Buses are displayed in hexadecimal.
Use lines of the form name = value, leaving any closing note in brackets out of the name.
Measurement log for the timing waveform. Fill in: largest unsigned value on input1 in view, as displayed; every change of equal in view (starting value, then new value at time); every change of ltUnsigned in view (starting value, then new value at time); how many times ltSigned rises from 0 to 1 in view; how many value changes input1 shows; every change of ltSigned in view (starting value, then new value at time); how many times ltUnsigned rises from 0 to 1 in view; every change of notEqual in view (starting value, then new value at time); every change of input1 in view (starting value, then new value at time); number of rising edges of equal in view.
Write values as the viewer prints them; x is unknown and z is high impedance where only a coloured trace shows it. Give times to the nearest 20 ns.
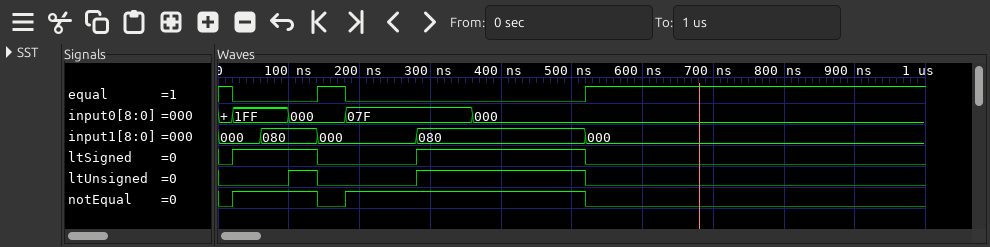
largest unsigned value on input1 in view, as displayed = 080
every change of equal in view = 1, 0 at 20 ns, 1 at 140 ns, 0 at 180 ns, 1 at 520 ns
every change of ltUnsigned in view = 0, 1 at 100 ns, 0 at 140 ns, 1 at 280 ns, 0 at 520 ns
how many times ltSigned rises from 0 to 1 in view = 2
how many value changes input1 shows = 4
every change of ltSigned in view = 0, 1 at 20 ns, 0 at 140 ns, 1 at 280 ns, 0 at 520 ns
how many times ltUnsigned rises from 0 to 1 in view = 2
every change of notEqual in view = 0, 1 at 20 ns, 0 at 140 ns, 1 at 180 ns, 0 at 520 ns
every change of input1 in view = 000, 080 at 60 ns, 000 at 140 ns, 080 at 280 ns, 000 at 520 ns
number of rising edges of equal in view = 2
